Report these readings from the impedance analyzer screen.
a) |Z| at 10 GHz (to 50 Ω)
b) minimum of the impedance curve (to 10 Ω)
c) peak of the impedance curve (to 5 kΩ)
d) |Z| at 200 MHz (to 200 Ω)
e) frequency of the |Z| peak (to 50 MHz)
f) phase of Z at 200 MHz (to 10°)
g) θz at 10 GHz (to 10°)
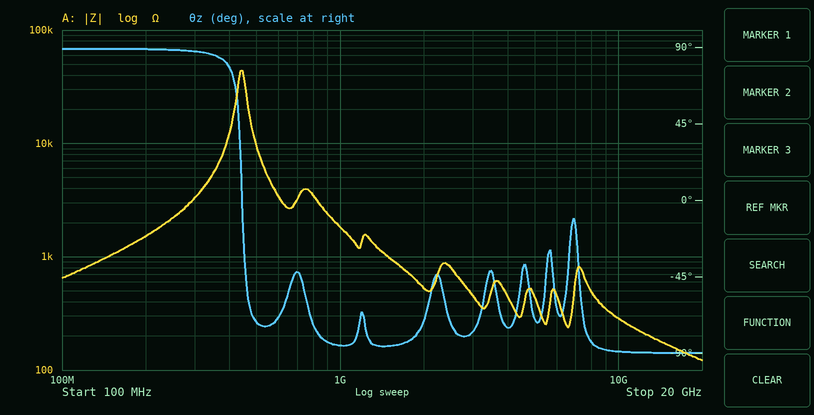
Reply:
300 Ω
120 Ω
45 kΩ
1.6 kΩ
450 MHz
90°
-90°
